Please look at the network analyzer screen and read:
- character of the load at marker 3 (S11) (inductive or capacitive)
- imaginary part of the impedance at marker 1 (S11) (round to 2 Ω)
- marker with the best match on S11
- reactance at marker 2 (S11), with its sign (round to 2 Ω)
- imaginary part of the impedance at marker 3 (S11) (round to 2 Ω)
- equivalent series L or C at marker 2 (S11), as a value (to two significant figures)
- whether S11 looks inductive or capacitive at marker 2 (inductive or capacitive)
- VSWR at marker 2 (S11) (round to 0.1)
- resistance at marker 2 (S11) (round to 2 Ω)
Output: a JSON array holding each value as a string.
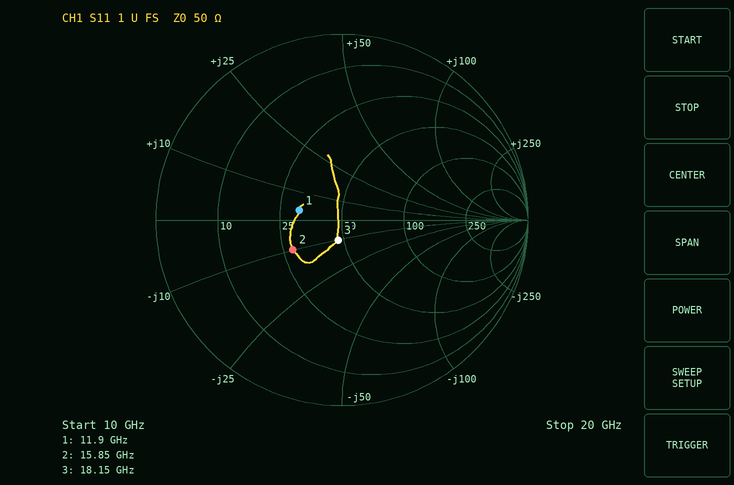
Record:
["capacitive", "+4 Ω", "marker 3", "-10 Ω", "-10 Ω", "1.0 pF", "capacitive", "1.9", "28 Ω"]
